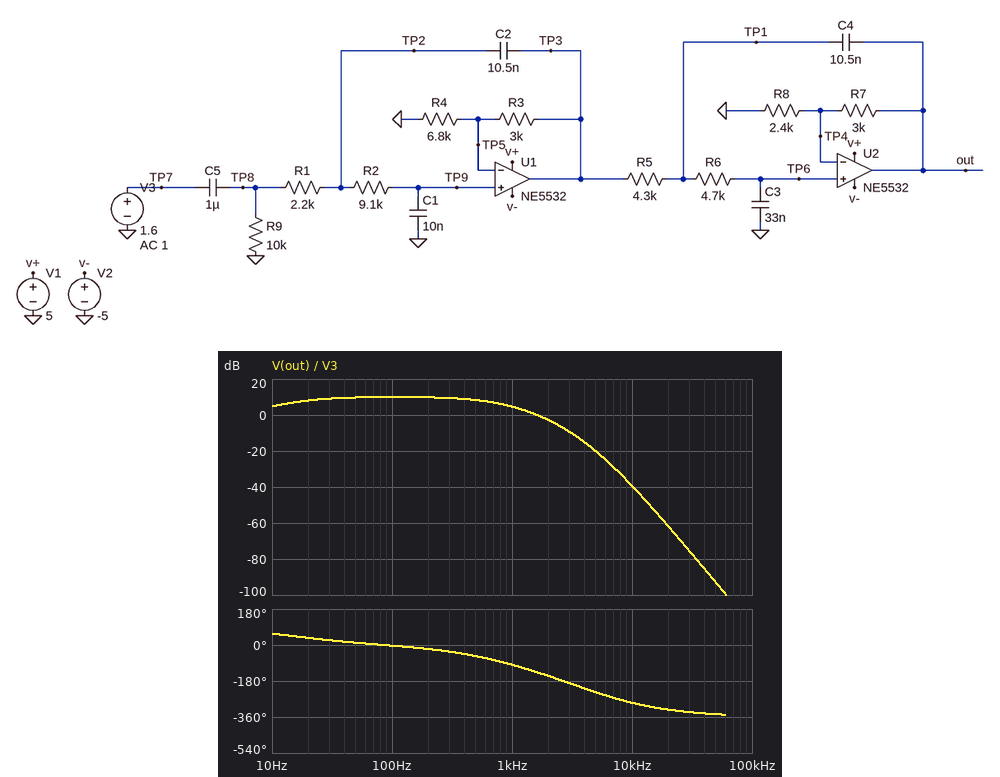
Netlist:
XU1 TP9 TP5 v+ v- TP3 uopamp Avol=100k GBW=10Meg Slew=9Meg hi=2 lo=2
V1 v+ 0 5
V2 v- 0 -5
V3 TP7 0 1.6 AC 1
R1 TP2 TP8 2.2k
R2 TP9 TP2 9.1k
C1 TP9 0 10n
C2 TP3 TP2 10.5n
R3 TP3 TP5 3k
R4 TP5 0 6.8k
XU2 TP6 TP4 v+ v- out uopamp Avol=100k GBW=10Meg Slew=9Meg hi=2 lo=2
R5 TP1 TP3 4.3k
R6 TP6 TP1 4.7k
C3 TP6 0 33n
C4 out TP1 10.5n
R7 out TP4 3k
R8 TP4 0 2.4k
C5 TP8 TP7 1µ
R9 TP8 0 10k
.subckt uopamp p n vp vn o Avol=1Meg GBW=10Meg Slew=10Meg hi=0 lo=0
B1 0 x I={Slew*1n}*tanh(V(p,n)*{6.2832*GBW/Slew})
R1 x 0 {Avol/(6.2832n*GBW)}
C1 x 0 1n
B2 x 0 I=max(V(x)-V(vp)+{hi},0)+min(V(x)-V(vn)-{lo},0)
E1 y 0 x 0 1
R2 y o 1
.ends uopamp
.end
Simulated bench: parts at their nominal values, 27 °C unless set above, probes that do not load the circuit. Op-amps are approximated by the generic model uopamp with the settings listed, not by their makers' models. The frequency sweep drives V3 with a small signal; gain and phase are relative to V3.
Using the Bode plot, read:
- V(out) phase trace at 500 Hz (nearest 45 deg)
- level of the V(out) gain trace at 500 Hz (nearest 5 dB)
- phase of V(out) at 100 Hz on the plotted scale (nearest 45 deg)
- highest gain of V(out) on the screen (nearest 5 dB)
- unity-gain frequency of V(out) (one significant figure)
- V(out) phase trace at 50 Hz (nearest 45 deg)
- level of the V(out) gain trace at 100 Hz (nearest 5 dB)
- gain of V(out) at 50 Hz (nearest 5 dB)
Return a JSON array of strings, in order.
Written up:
["-45 deg", "10 dB", "0 deg", "10 dB", "2 kHz", "0 deg", "10 dB", "10 dB"]
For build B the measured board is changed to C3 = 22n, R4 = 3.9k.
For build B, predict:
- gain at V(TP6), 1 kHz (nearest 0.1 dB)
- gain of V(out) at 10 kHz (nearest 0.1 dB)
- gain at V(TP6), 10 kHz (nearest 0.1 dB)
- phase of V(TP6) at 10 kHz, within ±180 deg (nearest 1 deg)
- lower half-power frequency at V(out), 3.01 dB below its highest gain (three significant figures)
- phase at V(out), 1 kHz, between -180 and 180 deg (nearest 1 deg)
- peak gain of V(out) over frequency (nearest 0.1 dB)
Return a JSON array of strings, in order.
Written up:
["2.5 dB", "-33.4 dB", "-40.4 dB", "67 deg", "15.5 Hz", "-80 deg", "11.9 dB"]
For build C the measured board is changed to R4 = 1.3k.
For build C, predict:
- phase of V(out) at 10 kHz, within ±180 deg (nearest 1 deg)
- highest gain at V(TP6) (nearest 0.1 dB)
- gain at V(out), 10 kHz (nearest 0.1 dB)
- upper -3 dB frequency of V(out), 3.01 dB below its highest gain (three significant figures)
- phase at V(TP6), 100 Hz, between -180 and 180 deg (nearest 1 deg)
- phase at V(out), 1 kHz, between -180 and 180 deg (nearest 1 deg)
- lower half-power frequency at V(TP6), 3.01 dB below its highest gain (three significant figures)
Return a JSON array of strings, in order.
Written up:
["57 deg", "10.3 dB", "-30.6 dB", "788 Hz", "-2 deg", "-86 deg", "15.5 Hz"]
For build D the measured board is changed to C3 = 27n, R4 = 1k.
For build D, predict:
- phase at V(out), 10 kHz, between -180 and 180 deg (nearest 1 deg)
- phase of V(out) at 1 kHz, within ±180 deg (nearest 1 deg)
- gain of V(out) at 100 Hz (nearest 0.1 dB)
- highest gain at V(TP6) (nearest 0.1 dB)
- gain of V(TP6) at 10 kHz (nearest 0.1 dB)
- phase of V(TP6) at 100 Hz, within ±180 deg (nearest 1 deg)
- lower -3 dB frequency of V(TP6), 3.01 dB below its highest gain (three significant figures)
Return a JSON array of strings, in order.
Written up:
["49 deg", "-73 deg", "19.1 dB", "12.1 dB", "-33.7 dB", "1 deg", "15.8 Hz"]
